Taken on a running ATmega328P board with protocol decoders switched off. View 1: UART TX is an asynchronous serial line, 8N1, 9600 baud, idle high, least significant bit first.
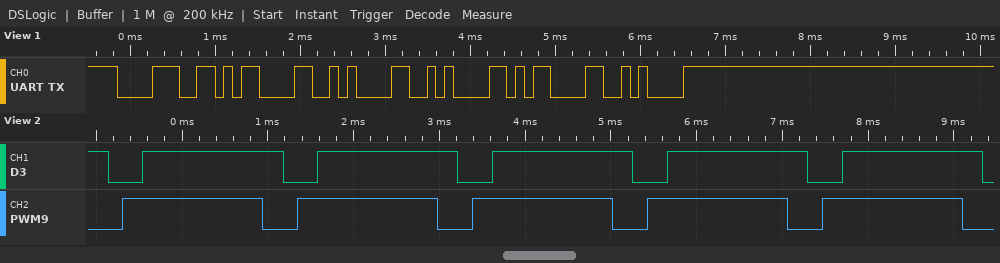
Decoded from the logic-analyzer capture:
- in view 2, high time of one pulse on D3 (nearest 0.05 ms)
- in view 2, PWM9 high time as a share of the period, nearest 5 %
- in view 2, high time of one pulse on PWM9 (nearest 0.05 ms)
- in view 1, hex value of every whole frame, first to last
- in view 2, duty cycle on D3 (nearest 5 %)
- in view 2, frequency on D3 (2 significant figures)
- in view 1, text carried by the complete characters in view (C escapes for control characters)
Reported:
1.65 ms
80 %
1.65 ms
38 0D 0A 0A 0D 0A
80 %
490 Hz
"8\r\n\n\r\n"
